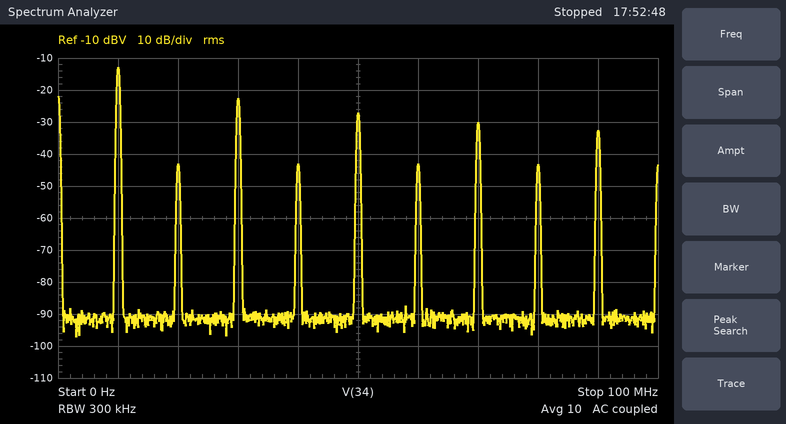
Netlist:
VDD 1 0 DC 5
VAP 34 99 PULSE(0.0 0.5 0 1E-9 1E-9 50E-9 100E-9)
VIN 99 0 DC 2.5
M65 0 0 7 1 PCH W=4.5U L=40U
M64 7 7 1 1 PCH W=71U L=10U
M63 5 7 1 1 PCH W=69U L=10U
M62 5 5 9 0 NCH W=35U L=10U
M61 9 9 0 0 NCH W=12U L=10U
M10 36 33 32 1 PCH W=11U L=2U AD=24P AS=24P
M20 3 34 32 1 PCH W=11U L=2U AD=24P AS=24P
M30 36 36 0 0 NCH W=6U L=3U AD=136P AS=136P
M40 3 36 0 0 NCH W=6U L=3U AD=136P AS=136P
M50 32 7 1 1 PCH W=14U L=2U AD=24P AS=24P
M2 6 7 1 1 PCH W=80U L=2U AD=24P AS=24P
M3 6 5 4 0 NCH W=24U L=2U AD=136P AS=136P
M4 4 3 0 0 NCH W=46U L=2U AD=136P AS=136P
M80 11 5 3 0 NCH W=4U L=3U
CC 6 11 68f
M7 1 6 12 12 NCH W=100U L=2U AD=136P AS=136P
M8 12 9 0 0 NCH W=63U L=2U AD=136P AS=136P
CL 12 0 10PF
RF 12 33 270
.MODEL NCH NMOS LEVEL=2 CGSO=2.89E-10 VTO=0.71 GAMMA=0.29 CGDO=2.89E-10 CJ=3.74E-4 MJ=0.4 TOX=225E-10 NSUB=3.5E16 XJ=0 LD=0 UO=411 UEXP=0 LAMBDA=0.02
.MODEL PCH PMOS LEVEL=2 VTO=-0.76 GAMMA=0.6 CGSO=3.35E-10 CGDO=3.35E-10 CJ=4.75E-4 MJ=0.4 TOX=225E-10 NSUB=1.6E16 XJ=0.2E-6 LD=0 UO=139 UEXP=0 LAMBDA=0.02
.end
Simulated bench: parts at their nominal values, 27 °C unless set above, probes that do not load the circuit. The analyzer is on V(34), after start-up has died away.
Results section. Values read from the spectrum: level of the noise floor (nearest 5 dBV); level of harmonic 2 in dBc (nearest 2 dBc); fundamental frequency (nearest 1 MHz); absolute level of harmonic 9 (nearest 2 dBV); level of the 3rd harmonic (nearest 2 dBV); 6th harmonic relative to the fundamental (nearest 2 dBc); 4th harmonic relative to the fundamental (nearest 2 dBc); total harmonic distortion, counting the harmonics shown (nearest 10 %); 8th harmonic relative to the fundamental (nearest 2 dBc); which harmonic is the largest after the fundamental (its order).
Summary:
-90 dBV
-30 dBc
10 MHz
-32 dBV
-22 dBV
-30 dBc
-30 dBc
40 %
-30 dBc
3
